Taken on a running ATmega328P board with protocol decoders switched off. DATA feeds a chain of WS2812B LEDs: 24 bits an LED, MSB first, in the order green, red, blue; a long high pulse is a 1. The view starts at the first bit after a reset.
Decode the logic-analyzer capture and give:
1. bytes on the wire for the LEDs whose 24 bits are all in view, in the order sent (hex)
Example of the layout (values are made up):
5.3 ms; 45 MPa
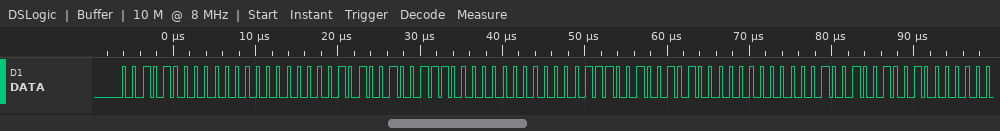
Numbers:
28 00 05 27 00 07 25 00 09
